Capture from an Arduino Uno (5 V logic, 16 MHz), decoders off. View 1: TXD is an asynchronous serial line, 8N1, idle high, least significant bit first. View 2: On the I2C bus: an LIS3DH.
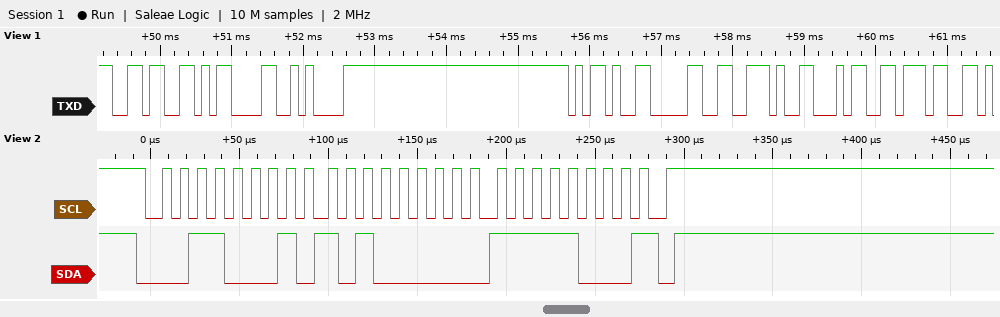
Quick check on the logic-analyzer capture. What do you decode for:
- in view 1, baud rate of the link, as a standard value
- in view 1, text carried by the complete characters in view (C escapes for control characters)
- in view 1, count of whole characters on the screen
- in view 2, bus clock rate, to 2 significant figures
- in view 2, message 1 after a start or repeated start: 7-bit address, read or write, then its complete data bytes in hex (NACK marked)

9600 baud
"6\r\n-0.47"
8
100 kHz
0x18 read: A0 F8 NACK
